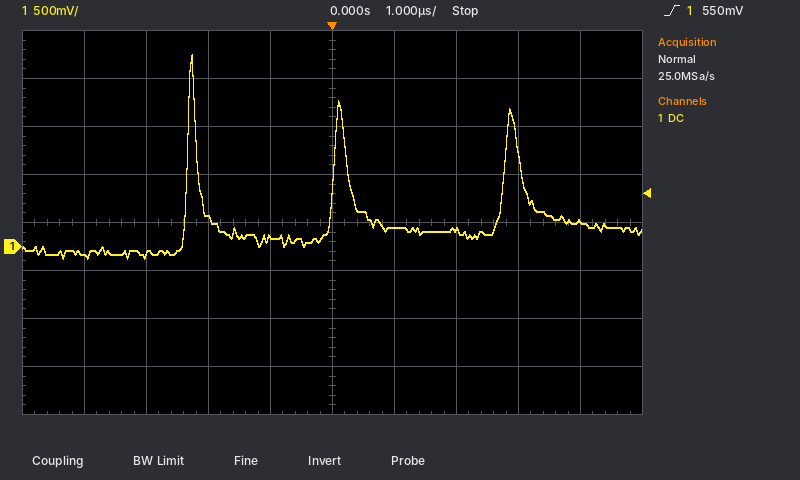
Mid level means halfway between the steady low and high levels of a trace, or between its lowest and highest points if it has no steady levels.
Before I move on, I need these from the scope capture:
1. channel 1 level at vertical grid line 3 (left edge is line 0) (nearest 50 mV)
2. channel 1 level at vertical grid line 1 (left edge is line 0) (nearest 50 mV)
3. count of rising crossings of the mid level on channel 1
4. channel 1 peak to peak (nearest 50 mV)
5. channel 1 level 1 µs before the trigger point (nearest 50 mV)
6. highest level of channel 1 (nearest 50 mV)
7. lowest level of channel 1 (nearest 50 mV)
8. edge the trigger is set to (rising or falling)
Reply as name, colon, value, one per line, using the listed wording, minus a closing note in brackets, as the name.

channel 1 level at vertical grid line 3 (left edge is line 0): 300 mV
channel 1 level at vertical grid line 1 (left edge is line 0): -100 mV
count of rising crossings of the mid level on channel 1: 3
channel 1 peak to peak: 2.10 V
channel 1 level 1 µs before the trigger point: 100 mV
highest level of channel 1: 2.00 V
lowest level of channel 1: -100 mV
edge the trigger is set to: rising
